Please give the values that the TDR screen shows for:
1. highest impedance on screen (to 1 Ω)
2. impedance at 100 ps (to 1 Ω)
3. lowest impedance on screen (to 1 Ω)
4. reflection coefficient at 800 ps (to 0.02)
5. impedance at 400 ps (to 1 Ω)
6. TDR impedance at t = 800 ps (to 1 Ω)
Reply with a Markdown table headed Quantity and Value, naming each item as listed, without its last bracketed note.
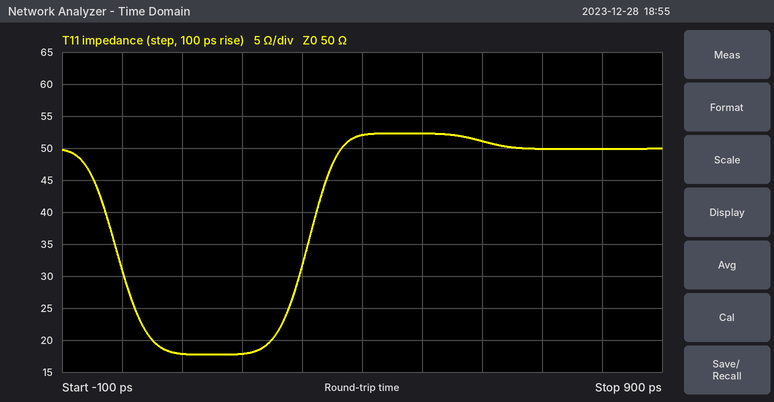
| Quantity | Value |
|---|---|
| highest impedance on screen | 52 Ω |
| impedance at 100 ps | 18 Ω |
| lowest impedance on screen | 18 Ω |
| reflection coefficient at 800 ps | 0.00 |
| impedance at 400 ps | 52 Ω |
| TDR impedance at t = 800 ps | 50 Ω |
